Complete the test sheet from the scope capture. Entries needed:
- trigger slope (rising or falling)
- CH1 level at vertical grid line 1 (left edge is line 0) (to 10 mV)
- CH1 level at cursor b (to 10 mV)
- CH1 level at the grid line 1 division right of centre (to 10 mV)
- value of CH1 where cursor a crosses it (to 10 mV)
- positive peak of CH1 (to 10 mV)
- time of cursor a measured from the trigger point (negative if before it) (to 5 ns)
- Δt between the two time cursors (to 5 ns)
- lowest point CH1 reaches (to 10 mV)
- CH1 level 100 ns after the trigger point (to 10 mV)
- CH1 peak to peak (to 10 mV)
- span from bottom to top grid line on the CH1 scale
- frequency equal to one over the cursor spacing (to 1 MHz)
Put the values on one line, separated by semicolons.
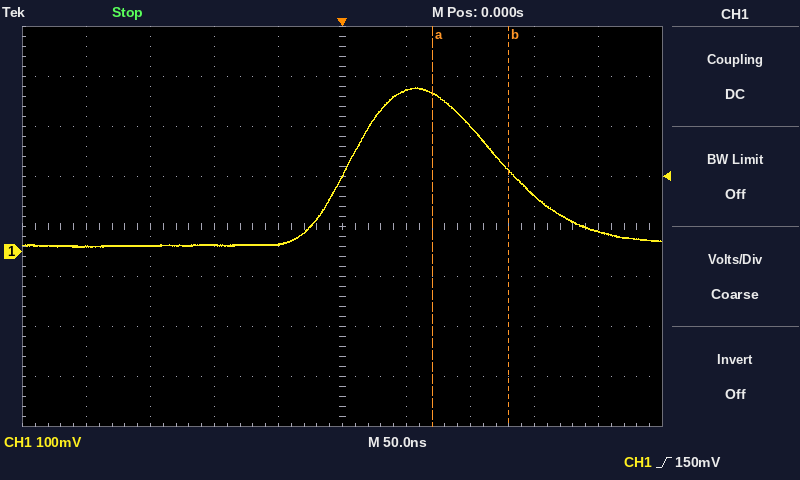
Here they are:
rising; 10 mV; 160 mV; 320 mV; 320 mV; 330 mV; +70 ns; 60 ns; 10 mV; 250 mV; 320 mV; 800 mV; 17 MHz
